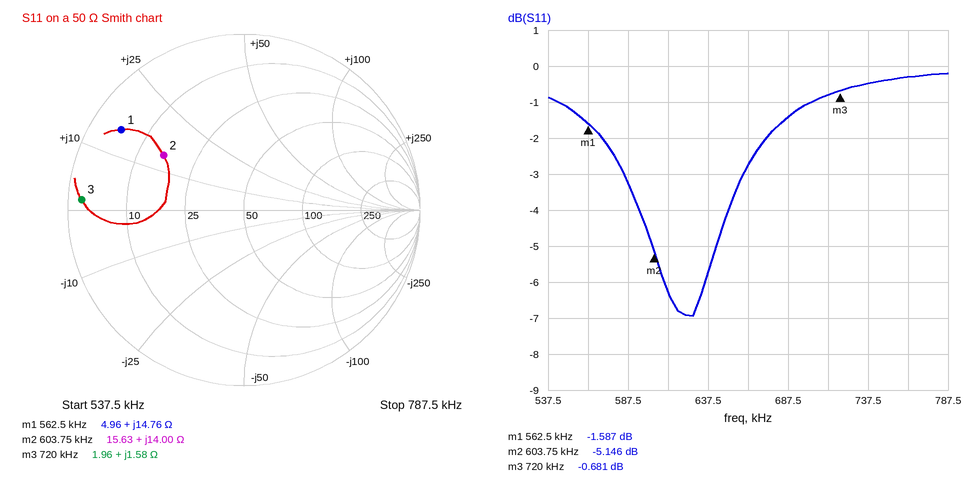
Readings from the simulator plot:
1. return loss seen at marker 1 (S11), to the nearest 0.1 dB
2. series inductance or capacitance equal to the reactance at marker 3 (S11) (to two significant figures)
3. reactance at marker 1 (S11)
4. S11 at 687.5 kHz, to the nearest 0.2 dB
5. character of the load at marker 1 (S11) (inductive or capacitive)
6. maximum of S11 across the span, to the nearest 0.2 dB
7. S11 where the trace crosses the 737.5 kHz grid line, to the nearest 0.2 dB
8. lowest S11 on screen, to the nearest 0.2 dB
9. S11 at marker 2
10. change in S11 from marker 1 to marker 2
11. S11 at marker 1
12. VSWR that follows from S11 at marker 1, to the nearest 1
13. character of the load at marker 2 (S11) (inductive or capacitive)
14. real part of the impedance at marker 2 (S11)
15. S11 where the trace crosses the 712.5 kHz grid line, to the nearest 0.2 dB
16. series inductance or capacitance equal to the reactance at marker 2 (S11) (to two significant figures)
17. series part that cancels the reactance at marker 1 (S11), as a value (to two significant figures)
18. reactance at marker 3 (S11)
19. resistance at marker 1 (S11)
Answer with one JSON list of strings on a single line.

["1.6 dB", "350 nH", "+14.76 Ω", "-1.4 dB", "inductive", "-0.2 dB", "-0.4 dB", "-7.0 dB", "-5.146 dB", "-3.559 dB", "-1.587 dB", "11", "inductive", "15.63 Ω", "-0.8 dB", "3.7 µH", "19 nF", "+1.58 Ω", "4.96 Ω"]
